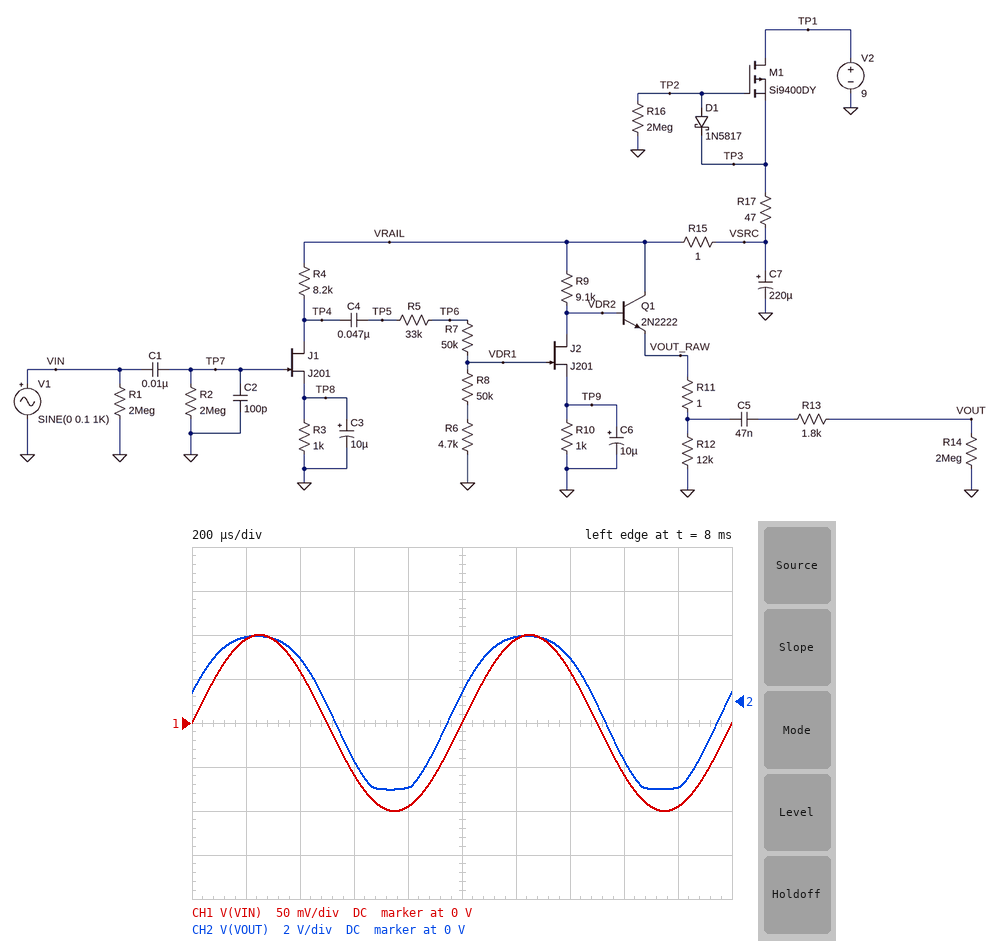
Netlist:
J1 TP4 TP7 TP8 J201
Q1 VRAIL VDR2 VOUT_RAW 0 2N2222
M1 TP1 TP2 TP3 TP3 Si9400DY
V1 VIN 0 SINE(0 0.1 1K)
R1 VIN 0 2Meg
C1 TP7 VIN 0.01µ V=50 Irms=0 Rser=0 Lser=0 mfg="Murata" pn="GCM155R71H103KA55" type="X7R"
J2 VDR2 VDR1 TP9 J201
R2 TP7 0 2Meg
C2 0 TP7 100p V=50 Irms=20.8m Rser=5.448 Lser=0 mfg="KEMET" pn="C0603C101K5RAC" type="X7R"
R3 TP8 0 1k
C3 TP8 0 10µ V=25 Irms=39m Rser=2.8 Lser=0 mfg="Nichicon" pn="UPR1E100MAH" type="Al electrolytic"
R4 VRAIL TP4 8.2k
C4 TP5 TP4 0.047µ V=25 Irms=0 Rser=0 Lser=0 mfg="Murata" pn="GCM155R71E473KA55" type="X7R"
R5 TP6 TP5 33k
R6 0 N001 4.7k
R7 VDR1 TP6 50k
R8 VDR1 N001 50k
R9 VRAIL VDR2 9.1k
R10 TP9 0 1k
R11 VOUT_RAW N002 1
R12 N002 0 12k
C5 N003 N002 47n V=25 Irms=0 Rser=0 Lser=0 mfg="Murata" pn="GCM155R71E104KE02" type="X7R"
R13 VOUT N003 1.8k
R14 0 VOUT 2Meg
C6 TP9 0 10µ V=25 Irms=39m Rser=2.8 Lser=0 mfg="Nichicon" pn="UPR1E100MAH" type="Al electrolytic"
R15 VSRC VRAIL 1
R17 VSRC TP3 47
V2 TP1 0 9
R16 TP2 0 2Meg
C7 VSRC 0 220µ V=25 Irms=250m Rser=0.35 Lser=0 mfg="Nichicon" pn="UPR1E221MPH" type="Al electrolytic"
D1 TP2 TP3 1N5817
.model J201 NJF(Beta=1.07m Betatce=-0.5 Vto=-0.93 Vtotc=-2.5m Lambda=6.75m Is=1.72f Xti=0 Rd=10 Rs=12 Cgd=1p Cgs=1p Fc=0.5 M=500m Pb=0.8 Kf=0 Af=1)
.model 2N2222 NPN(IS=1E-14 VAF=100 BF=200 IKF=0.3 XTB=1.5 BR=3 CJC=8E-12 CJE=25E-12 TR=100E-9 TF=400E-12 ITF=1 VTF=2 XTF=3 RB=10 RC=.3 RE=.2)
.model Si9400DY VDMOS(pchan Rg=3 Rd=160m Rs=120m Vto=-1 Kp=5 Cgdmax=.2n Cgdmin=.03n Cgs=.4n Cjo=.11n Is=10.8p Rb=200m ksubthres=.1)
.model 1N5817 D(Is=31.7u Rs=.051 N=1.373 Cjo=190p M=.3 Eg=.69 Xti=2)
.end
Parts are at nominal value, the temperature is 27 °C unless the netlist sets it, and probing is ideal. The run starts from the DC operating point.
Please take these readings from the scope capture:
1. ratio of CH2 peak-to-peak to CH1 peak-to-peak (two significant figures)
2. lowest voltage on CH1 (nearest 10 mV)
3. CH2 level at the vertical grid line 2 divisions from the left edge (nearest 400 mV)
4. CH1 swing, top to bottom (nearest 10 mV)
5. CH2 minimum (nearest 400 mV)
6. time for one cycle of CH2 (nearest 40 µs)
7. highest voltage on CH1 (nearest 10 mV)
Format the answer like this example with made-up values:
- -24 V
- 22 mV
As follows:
- 35
- -100 mV
- 2.0 V
- 200 mV
- -4.0 V
- 1.00 ms
- 100 mV
